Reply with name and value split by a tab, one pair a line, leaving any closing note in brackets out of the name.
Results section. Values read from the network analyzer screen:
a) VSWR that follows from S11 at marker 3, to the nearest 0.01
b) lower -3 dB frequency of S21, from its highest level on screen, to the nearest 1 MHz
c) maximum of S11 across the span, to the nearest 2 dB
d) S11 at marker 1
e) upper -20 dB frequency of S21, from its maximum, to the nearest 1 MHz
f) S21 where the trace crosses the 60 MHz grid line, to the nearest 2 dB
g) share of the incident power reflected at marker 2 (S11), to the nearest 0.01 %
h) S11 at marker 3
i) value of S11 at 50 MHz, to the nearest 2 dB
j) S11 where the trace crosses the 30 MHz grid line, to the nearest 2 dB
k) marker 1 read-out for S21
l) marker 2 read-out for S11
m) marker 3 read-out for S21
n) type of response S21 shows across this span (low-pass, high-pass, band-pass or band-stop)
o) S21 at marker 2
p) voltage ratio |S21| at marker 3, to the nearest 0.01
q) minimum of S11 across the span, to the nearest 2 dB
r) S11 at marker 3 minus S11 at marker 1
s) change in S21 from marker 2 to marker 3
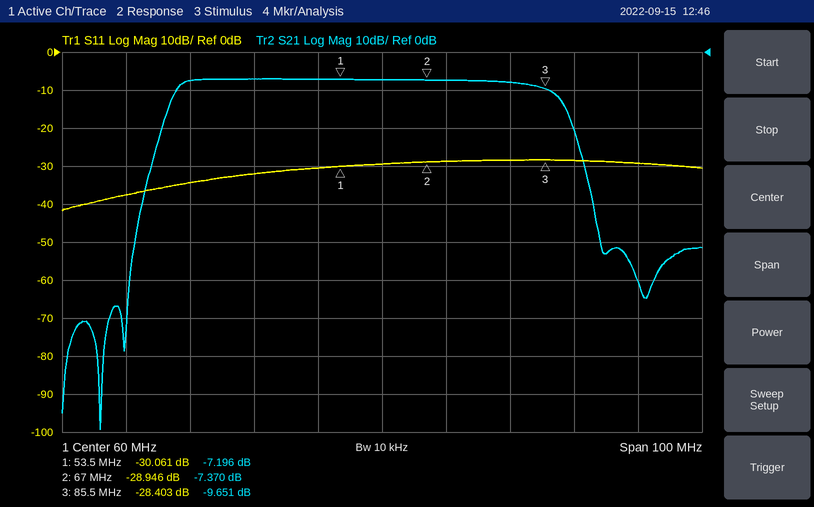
VSWR that follows from S11 at marker 3, to the nearest 0.01	1.08
lower -3 dB frequency of S21, from its highest level on screen, to the nearest 1 MHz	28 MHz
maximum of S11 across the span, to the nearest 2 dB	-28 dB
S11 at marker 1	-30.061 dB
upper -20 dB frequency of S21, from its maximum, to the nearest 1 MHz	91 MHz
S21 where the trace crosses the 60 MHz grid line, to the nearest 2 dB	-8 dB
share of the incident power reflected at marker 2 (S11), to the nearest 0.01 %	0.13 %
S11 at marker 3	-28.403 dB
value of S11 at 50 MHz, to the nearest 2 dB	-30 dB
S11 where the trace crosses the 30 MHz grid line, to the nearest 2 dB	-34 dB
marker 1 read-out for S21	-7.196 dB
marker 2 read-out for S11	-28.946 dB
marker 3 read-out for S21	-9.651 dB
type of response S21 shows across this span	band-pass
S21 at marker 2	-7.370 dB
voltage ratio |S21| at marker 3, to the nearest 0.01	0.33
minimum of S11 across the span, to the nearest 2 dB	-42 dB
S11 at marker 3 minus S11 at marker 1	1.658 dB
change in S21 from marker 2 to marker 3	-2.281 dB
